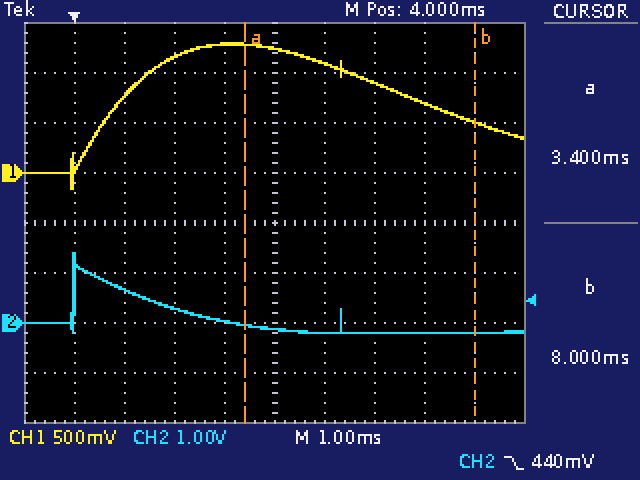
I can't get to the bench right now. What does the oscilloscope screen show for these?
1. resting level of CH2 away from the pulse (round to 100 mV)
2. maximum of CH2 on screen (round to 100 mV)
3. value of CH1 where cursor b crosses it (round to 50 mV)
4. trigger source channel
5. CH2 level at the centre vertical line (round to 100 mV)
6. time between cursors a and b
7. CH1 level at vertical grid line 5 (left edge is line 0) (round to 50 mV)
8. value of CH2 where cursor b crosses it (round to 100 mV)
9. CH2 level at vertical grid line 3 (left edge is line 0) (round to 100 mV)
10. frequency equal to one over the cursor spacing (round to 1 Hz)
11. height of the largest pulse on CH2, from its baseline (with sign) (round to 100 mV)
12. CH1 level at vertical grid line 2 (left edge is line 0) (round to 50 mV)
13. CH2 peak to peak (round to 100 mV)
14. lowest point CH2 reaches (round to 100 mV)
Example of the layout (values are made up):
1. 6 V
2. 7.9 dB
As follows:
1. -200 mV
2. 1.4 V
3. 500 mV
4. CH2
5. -100 mV
6. 4.6 ms
7. 1.25 V
8. -200 mV
9. 300 mV
10. 217 Hz
11. +1.6 V
12. 750 mV
13. 1.6 V
14. -200 mV
